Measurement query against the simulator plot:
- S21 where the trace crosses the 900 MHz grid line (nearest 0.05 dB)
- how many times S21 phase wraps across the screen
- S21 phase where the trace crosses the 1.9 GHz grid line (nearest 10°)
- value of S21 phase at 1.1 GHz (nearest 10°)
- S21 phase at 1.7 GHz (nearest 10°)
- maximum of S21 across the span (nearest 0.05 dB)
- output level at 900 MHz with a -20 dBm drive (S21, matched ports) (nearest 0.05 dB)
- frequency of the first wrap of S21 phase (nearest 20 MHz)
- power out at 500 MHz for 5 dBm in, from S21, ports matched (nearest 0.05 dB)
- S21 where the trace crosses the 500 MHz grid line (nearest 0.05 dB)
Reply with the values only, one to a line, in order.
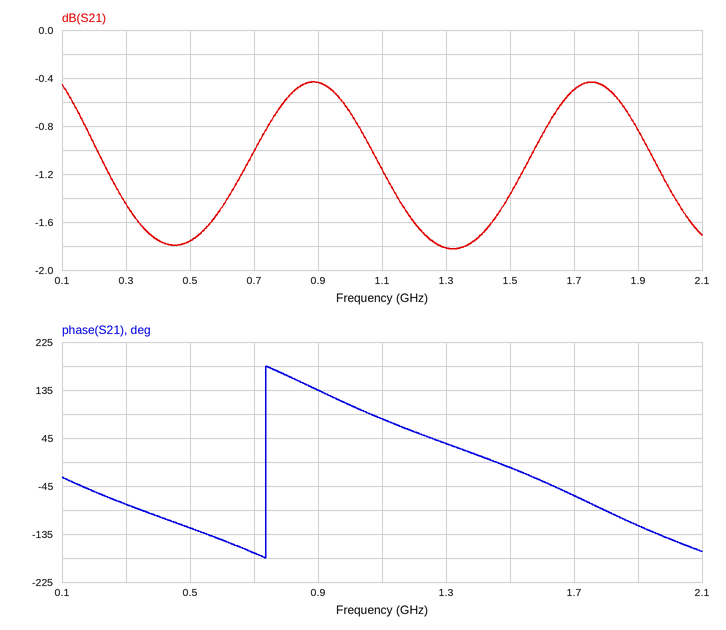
-0.45 dB
1
-120°
80°
-60°
-0.45 dB
-20.45 dBm
740 MHz
3.25 dBm
-1.75 dB
